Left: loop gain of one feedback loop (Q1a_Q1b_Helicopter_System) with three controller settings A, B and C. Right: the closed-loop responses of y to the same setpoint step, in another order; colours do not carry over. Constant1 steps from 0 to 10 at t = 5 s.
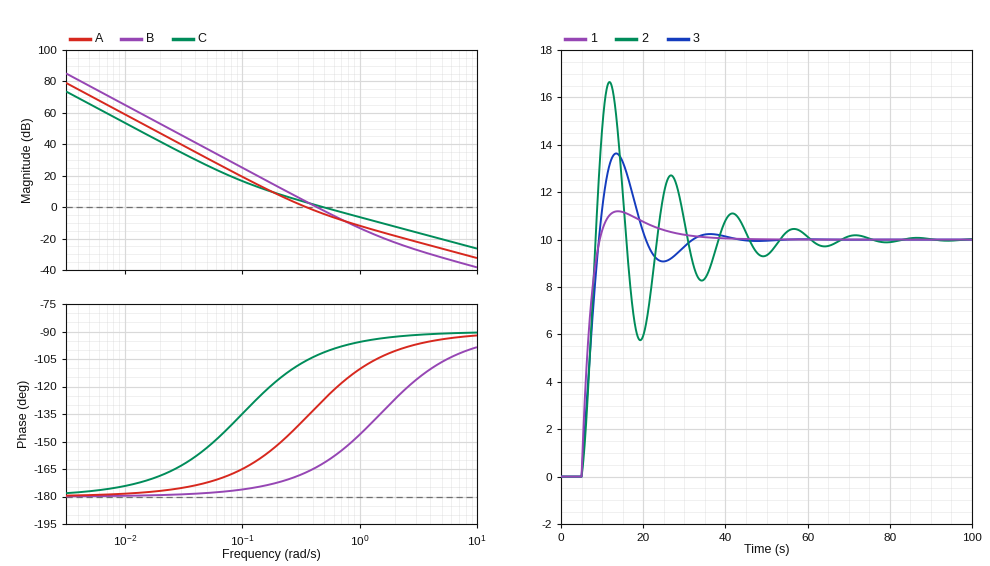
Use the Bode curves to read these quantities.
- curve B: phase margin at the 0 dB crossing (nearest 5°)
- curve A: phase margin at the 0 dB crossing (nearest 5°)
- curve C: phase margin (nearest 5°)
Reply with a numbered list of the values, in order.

1. 15°
2. 45°
3. 80°
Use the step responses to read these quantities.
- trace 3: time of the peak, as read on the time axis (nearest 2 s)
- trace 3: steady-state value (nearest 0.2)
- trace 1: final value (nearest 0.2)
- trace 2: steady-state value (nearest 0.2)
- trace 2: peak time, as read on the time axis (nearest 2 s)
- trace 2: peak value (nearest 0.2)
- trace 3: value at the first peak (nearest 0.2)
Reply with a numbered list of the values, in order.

1. 14 s
2. 10.0
3. 10.0
4. 10.0
5. 12 s
6. 16.6
7. 13.6
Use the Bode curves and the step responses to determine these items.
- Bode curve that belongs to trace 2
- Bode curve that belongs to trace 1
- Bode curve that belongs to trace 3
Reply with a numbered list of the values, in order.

1. B
2. C
3. A
